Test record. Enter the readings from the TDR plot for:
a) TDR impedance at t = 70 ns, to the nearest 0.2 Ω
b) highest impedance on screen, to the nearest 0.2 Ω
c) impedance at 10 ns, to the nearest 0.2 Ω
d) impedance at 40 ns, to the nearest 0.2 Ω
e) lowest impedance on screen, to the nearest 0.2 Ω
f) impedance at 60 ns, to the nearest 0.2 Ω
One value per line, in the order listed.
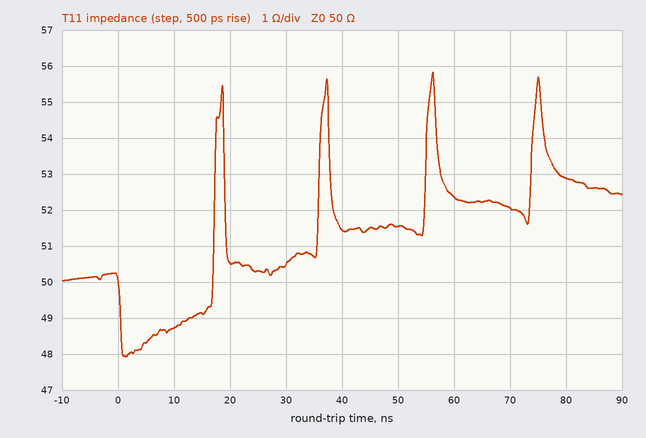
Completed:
52.0 Ω
55.8 Ω
48.8 Ω
51.4 Ω
48.0 Ω
52.4 Ω
